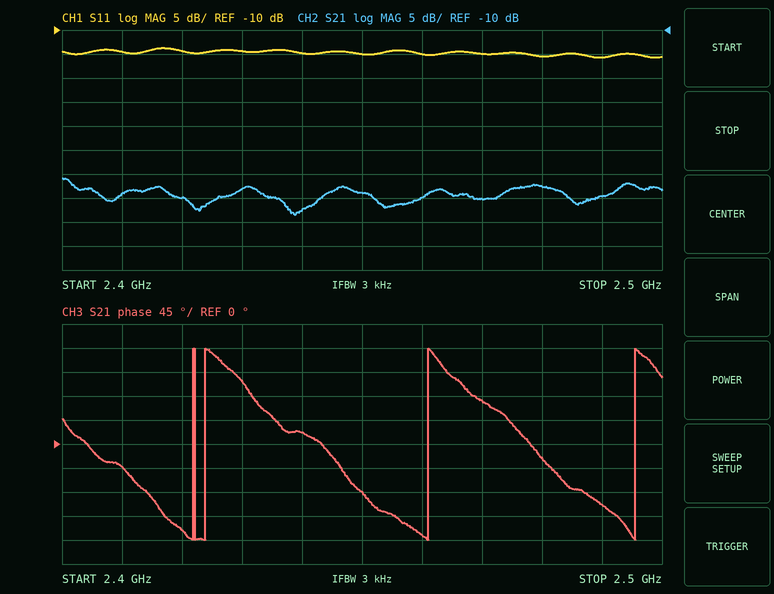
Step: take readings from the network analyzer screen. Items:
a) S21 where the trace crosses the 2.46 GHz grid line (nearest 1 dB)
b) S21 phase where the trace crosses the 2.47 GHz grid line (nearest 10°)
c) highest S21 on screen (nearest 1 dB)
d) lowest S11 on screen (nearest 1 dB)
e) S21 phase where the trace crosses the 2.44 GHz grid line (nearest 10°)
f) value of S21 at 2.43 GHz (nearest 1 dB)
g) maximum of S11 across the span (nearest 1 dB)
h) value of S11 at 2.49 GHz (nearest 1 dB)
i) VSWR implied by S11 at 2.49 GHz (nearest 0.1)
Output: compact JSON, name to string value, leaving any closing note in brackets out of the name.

{"S21 where the trace crosses the 2.46 GHz grid line": "-45 dB", "S21 phase where the trace crosses the 2.47 GHz grid line": "80°", "highest S21 on screen": "-41 dB", "lowest S11 on screen": "-16 dB", "S21 phase where the trace crosses the 2.44 GHz grid line": "20°", "value of S21 at 2.43 GHz": "-43 dB", "maximum of S11 across the span": "-14 dB", "value of S11 at 2.49 GHz": "-16 dB", "VSWR implied by S11 at 2.49 GHz": "1.4"}
